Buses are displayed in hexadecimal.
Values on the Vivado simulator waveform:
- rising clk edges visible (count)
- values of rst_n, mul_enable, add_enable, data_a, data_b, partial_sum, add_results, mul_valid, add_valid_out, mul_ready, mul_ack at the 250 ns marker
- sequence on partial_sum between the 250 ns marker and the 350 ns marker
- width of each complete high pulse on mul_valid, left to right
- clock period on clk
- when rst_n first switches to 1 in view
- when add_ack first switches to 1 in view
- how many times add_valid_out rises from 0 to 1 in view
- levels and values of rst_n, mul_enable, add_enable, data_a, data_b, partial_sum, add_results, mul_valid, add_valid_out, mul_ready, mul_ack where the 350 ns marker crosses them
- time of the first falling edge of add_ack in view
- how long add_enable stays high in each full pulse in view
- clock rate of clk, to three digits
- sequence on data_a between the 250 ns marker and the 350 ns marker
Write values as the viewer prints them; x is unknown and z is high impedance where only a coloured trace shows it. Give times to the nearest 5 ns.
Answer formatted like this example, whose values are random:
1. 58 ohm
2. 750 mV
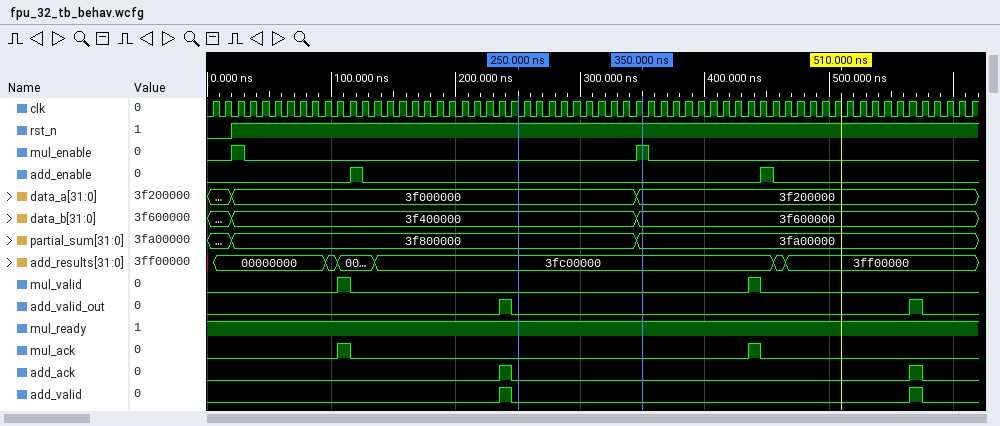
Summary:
1. 62
2. rst_n=1, mul_enable=0, add_enable=0, data_a=3f000000, data_b=3f400000, partial_sum=3f800000, add_results=3fc00000, mul_valid=0, add_valid_out=0, mul_ready=1, mul_ack=0
3. 3f800000, 3fa00000
4. 10 ns, 10 ns
5. 10 ns
6. 20 ns
7. 235 ns
8. 2
9. rst_n=1, mul_enable=1, add_enable=0, data_a=3f200000, data_b=3f600000, partial_sum=3fa00000, add_results=3fc00000, mul_valid=0, add_valid_out=0, mul_ready=1, mul_ack=0
10. 245 ns
11. 10 ns, 10 ns
12. 100 MHz
13. 3f000000, 3f200000
